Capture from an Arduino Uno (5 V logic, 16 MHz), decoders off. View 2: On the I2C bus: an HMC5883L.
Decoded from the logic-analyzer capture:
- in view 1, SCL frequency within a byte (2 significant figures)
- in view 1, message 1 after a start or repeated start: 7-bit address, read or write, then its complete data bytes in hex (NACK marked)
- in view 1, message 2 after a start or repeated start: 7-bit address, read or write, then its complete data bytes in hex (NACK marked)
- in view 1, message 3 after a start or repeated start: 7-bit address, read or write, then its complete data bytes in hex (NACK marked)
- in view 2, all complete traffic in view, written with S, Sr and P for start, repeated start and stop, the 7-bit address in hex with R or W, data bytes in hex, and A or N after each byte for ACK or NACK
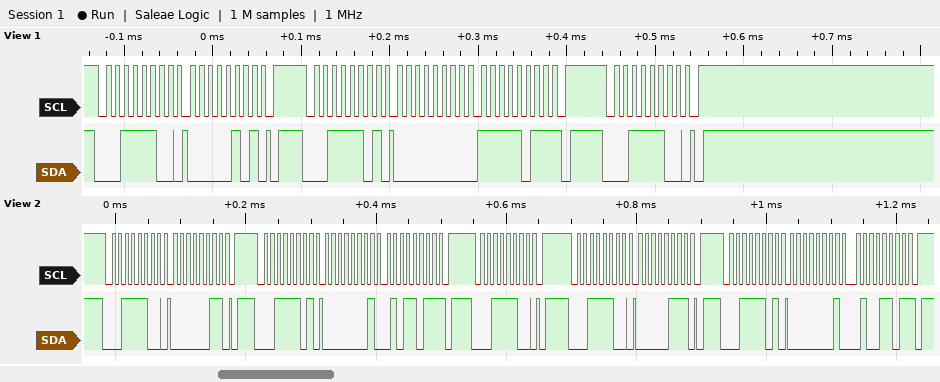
100 kHz
0x1E write: 05
0x1E read: 00 FB NACK
0x1E write
S 1EW A 03 A P S 1ER A 01 A 5B N P S 1EW A P S 1EW A 07 A P S 1ER A 01 A 4D N P
